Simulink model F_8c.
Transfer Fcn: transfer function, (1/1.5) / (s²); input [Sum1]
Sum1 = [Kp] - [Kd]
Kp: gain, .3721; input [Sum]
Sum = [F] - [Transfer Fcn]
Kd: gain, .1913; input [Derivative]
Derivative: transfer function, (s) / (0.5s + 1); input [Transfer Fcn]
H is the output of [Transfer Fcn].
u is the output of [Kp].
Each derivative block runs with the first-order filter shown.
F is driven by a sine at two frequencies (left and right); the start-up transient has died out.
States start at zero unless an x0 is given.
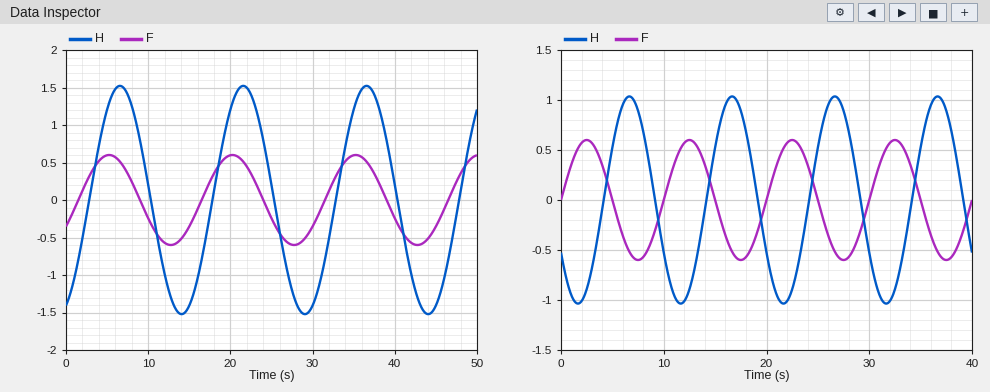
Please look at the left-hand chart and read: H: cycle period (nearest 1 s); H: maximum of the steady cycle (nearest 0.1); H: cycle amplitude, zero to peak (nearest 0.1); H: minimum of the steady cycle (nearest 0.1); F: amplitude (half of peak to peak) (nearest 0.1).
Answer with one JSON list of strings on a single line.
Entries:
["15 s", "1.5", "1.5", "-1.5", "0.6"]
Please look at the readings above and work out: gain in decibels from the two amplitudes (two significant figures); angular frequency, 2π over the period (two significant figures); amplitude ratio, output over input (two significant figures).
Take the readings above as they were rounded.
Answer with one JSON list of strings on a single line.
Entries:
["8.0 dB", "0.42 rad/s", "2.5"]
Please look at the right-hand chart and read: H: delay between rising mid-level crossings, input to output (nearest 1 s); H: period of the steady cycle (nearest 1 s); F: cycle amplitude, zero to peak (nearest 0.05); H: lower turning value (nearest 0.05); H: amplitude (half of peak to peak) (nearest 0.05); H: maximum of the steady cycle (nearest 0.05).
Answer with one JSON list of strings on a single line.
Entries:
["4 s", "10 s", "0.60", "-1.05", "1.05", "1.05"]
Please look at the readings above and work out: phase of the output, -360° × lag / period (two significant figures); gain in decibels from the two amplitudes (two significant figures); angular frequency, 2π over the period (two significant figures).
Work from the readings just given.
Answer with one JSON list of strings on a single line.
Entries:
["-140°", "4.9 dB", "0.63 rad/s"]
